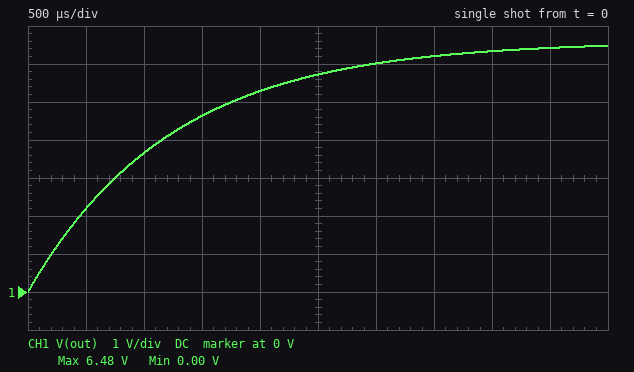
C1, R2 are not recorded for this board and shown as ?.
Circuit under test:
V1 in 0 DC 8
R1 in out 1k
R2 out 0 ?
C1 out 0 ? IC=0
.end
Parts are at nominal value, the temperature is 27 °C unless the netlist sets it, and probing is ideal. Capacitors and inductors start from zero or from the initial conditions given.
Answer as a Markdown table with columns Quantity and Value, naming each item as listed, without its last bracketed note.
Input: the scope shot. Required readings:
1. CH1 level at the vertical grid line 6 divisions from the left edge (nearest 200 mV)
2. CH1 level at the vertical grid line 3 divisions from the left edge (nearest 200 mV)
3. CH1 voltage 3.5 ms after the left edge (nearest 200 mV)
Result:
| Quantity | Value |
|---|---|
| CH1 level at the vertical grid line 6 divisions from the left edge | 6.0 V |
| CH1 level at the vertical grid line 3 divisions from the left edge | 4.6 V |
| CH1 voltage 3.5 ms after the left edge | 6.2 V |
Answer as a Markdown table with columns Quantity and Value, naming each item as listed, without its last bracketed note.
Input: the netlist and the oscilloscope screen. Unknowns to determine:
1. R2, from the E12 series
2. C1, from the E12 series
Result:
| Quantity | Value |
|---|---|
| R2, from the E12 series | 4.7 kΩ |
| C1, from the E12 series | 1.5 µF |
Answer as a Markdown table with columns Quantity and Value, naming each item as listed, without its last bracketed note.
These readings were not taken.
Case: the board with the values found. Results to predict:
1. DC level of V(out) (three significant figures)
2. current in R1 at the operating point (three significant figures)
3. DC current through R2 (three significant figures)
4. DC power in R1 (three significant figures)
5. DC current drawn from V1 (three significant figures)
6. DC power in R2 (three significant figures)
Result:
| Quantity | Value |
|---|---|
| DC level of V(out) | 6.60 V |
| current in R1 at the operating point | 1.40 mA |
| DC current through R2 | 1.40 mA |
| DC power in R1 | 1.97 mW |
| DC current drawn from V1 | 1.40 mA |
| DC power in R2 | 9.26 mW |
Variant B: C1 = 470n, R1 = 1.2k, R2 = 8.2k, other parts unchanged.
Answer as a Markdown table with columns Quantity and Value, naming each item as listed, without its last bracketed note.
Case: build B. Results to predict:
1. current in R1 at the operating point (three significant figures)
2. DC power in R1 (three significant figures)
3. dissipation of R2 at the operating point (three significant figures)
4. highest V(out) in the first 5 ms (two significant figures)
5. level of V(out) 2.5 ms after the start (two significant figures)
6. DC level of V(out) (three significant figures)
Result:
| Quantity | Value |
|---|---|
| current in R1 at the operating point | 851 µA |
| DC power in R1 | 869 µW |
| dissipation of R2 at the operating point | 5.94 mW |
| highest V(out) in the first 5 ms | 7.0 V |
| level of V(out) 2.5 ms after the start | 6.9 V |
| DC level of V(out) | 6.98 V |
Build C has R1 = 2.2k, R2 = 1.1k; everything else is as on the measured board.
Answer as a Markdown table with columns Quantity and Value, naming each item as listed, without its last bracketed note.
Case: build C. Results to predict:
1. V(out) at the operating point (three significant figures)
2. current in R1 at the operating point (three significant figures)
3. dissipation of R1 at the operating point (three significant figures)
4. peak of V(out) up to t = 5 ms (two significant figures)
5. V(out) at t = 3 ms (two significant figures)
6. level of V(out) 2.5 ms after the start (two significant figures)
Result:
| Quantity | Value |
|---|---|
| V(out) at the operating point | 2.67 V |
| current in R1 at the operating point | 2.42 mA |
| dissipation of R1 at the operating point | 12.9 mW |
| peak of V(out) up to t = 5 ms | 2.6 V |
| V(out) at t = 3 ms | 2.5 V |
| level of V(out) 2.5 ms after the start | 2.4 V |
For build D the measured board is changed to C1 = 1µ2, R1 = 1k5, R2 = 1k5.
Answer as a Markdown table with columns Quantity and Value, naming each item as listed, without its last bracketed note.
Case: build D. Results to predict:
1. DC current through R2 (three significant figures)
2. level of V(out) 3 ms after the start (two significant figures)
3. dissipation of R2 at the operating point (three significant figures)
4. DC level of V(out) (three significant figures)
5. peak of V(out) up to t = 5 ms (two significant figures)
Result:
| Quantity | Value |
|---|---|
| DC current through R2 | 2.67 mA |
| level of V(out) 3 ms after the start | 3.9 V |
| dissipation of R2 at the operating point | 10.7 mW |
| DC level of V(out) | 4.00 V |
| peak of V(out) up to t = 5 ms | 4.0 V |
